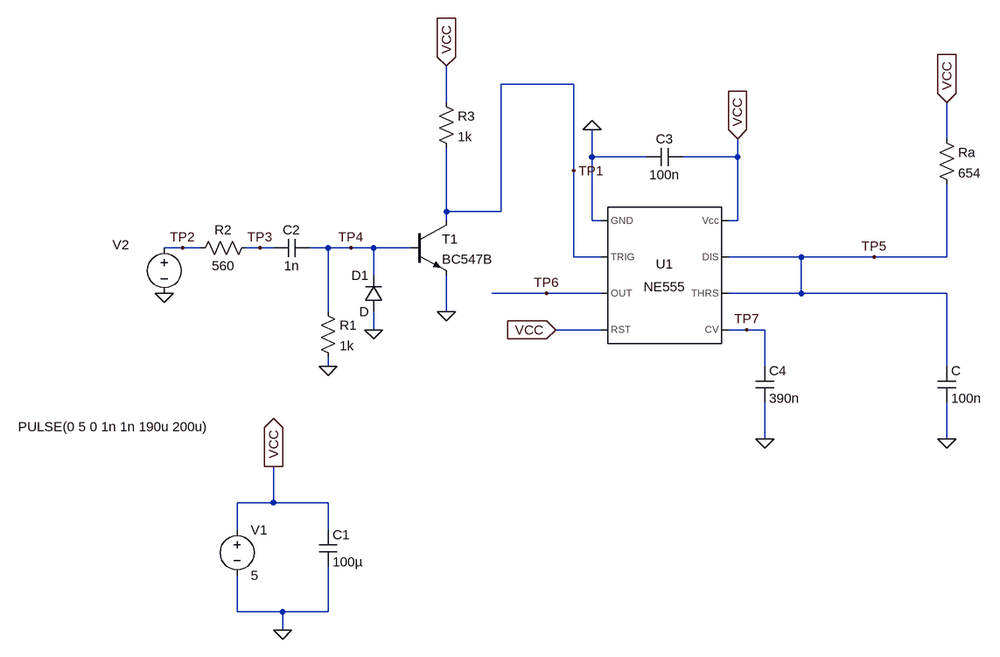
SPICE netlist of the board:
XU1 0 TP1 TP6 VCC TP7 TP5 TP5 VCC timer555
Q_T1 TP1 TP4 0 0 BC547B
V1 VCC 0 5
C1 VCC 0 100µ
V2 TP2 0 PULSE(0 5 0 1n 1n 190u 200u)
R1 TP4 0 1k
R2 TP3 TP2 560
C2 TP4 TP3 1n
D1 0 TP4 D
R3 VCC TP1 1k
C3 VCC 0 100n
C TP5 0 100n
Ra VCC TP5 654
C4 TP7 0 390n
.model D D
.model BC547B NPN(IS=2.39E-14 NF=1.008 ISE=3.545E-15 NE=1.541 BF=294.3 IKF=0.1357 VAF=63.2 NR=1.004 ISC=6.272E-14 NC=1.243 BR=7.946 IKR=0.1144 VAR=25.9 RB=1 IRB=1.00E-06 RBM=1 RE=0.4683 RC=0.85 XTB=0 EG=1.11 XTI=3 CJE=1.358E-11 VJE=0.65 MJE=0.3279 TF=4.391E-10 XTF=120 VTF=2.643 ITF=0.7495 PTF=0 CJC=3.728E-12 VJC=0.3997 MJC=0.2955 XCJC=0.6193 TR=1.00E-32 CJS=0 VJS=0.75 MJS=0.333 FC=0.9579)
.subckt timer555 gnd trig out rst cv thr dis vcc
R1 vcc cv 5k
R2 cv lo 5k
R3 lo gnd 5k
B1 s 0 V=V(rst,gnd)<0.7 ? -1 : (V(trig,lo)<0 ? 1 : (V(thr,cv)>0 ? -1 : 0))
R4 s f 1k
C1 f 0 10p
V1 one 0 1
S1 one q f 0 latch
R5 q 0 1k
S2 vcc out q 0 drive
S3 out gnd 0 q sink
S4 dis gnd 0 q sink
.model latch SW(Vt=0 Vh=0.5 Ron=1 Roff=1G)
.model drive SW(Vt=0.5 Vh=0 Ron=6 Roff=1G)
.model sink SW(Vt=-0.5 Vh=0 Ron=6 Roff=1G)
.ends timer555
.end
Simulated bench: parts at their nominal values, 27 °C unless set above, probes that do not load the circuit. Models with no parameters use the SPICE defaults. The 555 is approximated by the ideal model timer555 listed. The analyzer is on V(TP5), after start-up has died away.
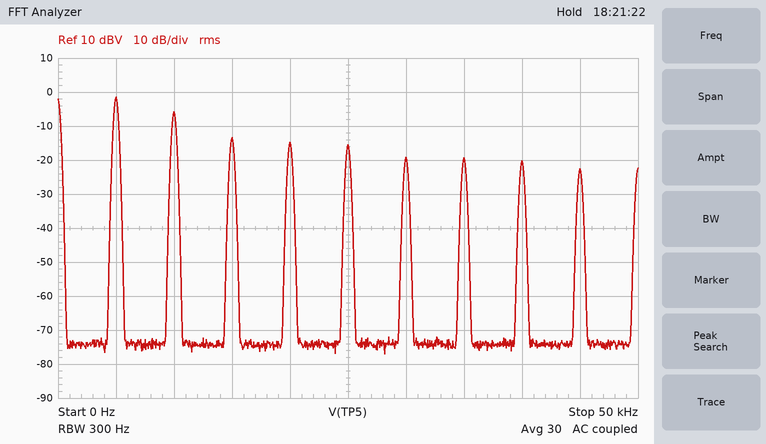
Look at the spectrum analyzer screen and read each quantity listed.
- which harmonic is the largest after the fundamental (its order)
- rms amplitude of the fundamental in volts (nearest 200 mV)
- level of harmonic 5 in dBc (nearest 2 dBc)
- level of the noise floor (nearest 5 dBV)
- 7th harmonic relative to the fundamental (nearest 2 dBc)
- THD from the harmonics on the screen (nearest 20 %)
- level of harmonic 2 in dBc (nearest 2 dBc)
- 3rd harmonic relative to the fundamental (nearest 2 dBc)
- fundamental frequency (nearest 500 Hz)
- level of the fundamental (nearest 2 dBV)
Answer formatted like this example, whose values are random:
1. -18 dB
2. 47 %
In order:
1. 2
2. 800 mV
3. -14 dBc
4. -75 dBV
5. -18 dBc
6. 80 %
7. -4 dBc
8. -12 dBc
9. 5.0 kHz
10. -2 dBV
